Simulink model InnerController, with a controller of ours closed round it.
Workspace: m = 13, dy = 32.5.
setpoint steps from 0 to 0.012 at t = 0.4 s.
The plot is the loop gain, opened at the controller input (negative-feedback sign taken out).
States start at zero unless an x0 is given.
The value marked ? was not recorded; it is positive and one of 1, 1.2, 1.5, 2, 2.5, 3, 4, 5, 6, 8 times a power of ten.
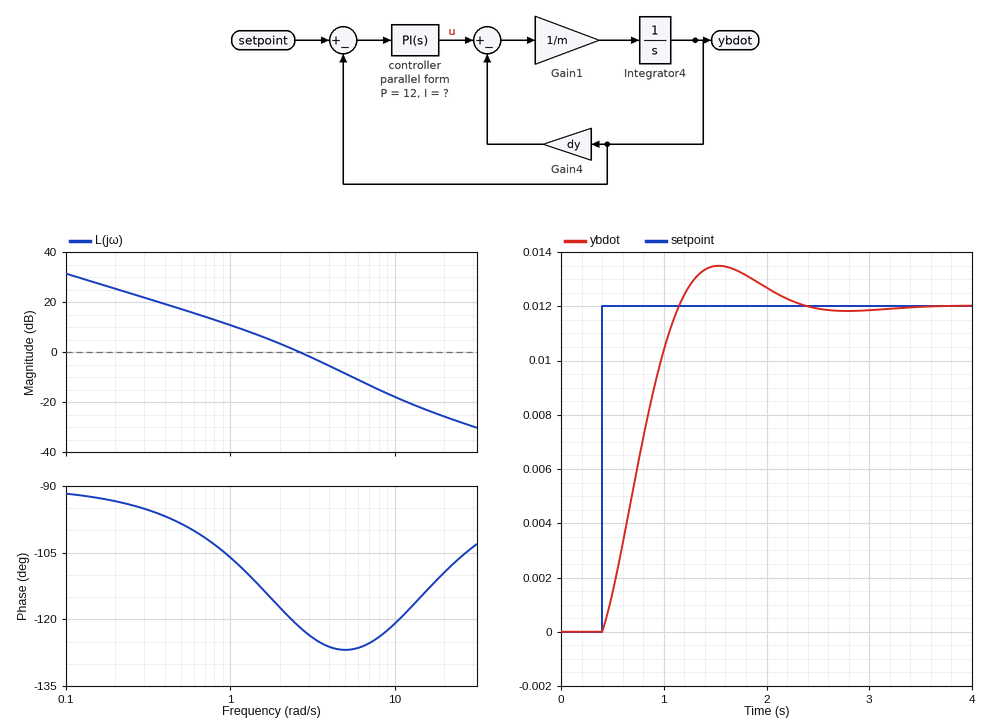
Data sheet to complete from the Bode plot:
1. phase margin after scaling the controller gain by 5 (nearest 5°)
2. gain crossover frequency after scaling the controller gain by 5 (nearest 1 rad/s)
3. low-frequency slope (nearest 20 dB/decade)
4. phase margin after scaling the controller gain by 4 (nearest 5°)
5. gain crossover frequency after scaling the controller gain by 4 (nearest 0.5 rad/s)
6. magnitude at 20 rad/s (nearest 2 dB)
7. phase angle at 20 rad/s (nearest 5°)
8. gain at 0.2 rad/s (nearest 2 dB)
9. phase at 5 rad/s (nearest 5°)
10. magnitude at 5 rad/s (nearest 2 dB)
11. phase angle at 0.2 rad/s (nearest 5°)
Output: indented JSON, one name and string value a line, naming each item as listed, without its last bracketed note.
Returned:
{
  "phase margin after scaling the controller gain by 5": "55°",
  "gain crossover frequency after scaling the controller gain by 5": "7 rad/s",
  "low-frequency slope": "-20 dB/decade",
  "phase margin after scaling the controller gain by 4": "55°",
  "gain crossover frequency after scaling the controller gain by 4": "6.5 rad/s",
  "magnitude at 20 rad/s": "-26 dB",
  "phase angle at 20 rad/s": "-110°",
  "gain at 0.2 rad/s": "26 dB",
  "phase at 5 rad/s": "-125°",
  "magnitude at 5 rad/s": "-8 dB",
  "phase angle at 0.2 rad/s": "-95°"
}
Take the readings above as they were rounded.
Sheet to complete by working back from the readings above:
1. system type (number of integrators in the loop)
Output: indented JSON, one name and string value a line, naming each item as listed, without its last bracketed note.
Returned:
{
  "system type": "1"
}
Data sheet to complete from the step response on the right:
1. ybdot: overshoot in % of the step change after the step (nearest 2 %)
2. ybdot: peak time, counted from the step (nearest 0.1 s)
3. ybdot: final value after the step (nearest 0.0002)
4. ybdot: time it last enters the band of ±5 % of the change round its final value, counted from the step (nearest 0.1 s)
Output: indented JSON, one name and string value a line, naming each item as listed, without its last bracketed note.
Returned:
{
  "ybdot: overshoot in % of the step change after the step": "12 %",
  "ybdot: peak time, counted from the step": "1.1 s",
  "ybdot: final value after the step": "0.0120",
  "ybdot: time it last enters the band of ±5 % of the change round its final value, counted from the step": "1.6 s"
}
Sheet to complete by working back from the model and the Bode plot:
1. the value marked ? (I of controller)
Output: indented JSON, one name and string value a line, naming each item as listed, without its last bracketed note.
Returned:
{
  "the value marked ?": "120"
}
